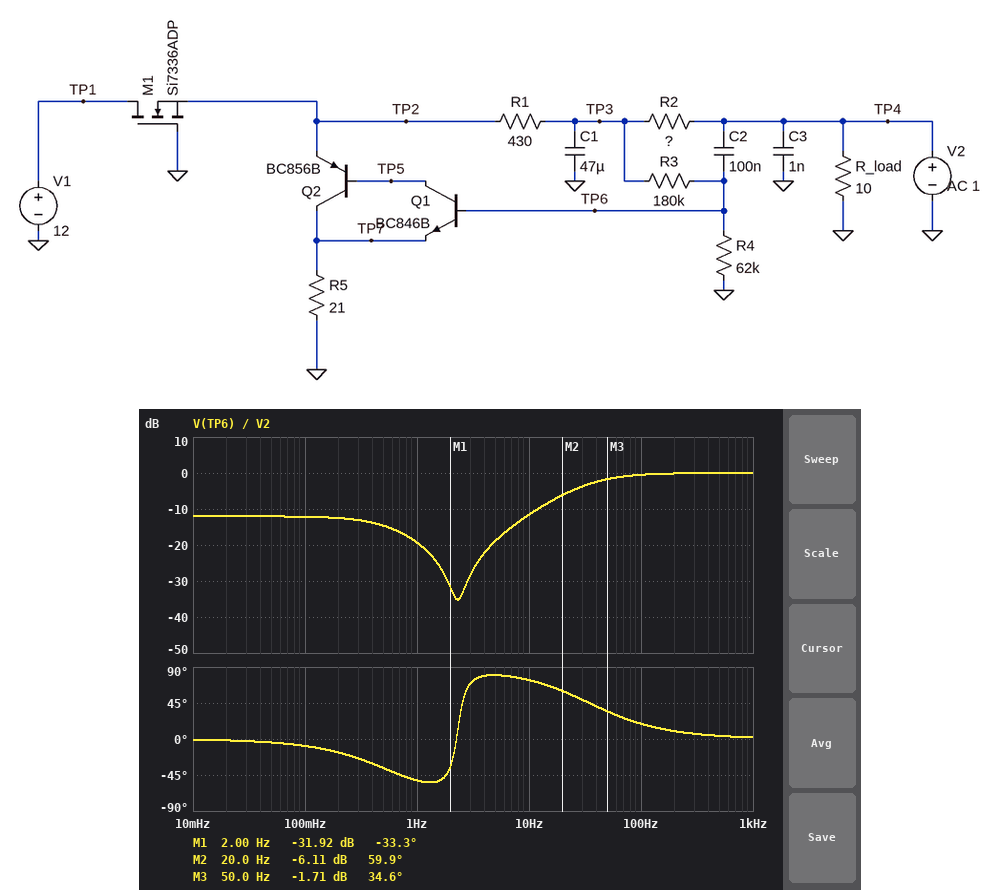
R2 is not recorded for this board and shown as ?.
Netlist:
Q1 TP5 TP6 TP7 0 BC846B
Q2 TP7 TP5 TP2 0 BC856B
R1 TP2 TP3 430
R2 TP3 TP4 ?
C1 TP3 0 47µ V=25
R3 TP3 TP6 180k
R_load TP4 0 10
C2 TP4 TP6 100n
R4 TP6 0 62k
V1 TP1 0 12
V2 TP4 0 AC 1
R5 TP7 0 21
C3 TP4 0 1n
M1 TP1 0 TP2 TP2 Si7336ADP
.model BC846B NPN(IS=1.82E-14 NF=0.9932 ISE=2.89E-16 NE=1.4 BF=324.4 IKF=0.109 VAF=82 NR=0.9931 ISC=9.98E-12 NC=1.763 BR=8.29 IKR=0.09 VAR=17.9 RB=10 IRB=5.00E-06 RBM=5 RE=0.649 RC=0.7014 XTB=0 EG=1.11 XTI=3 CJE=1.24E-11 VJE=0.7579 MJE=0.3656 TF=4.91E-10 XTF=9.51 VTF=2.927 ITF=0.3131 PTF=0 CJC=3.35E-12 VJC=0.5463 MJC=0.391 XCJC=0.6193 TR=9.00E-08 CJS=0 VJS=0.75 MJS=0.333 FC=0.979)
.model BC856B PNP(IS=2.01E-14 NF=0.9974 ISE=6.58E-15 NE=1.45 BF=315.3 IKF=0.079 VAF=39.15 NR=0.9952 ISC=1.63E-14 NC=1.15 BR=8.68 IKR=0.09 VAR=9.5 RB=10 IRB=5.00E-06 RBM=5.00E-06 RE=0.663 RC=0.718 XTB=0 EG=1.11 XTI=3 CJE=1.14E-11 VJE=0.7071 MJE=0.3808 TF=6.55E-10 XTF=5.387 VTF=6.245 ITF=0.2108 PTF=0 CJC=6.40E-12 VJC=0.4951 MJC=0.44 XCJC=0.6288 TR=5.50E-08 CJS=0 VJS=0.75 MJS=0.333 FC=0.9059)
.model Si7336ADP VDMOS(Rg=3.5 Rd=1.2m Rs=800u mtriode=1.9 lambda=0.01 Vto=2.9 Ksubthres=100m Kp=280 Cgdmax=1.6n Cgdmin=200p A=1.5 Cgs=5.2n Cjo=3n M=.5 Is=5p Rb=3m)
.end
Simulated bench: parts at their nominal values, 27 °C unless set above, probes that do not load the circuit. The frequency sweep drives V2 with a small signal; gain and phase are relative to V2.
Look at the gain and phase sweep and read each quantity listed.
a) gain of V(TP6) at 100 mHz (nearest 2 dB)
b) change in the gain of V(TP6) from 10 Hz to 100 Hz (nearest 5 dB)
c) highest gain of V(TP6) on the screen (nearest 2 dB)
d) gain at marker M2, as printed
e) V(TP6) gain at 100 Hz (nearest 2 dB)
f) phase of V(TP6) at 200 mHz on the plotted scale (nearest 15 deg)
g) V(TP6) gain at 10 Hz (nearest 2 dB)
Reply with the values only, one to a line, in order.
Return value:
-12 dB
10 dB
0 dB
-6.11 dB
0 dB
-15 deg
-12 dB
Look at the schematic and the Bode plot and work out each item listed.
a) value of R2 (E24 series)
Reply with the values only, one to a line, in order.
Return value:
5.6 kΩ
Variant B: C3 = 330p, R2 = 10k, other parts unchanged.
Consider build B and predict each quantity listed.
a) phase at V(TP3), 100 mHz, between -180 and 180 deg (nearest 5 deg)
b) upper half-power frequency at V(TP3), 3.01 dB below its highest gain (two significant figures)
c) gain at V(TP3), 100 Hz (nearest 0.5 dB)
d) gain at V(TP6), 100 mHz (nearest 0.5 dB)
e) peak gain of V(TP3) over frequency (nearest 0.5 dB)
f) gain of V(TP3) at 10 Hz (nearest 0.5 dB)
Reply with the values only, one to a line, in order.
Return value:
-15 deg
350 mHz
-49.0 dB
-12.5 dB
-0.5 dB
-29.5 dB
